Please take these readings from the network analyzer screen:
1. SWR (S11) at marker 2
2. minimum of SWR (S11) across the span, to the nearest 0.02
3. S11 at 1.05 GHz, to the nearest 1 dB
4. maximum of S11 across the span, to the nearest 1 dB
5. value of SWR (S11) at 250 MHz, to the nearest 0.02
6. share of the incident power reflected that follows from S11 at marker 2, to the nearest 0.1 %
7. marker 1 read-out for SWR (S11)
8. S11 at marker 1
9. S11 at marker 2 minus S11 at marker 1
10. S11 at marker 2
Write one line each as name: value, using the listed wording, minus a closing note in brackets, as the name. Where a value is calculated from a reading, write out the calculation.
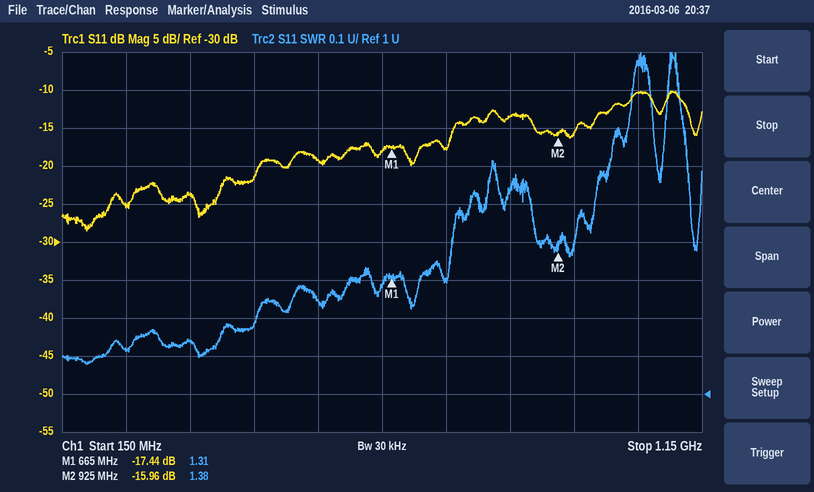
SWR (S11) at marker 2: 1.38
minimum of SWR (S11) across the span, to the nearest 0.02: 1.08
S11 at 1.05 GHz, to the nearest 1 dB: -10 dB
maximum of S11 across the span, to the nearest 1 dB: -10 dB
value of SWR (S11) at 250 MHz, to the nearest 0.02: 1.12
share of the incident power reflected that follows from S11 at marker 2, to the nearest 0.1 %: 10^(-15.96/10) ≈ 2.5 %
marker 1 read-out for SWR: 1.31
S11 at marker 1: -17.44 dB
S11 at marker 2 minus S11 at marker 1: -15.96 − (-17.44) = 1.48 dB
S11 at marker 2: -15.96 dB
